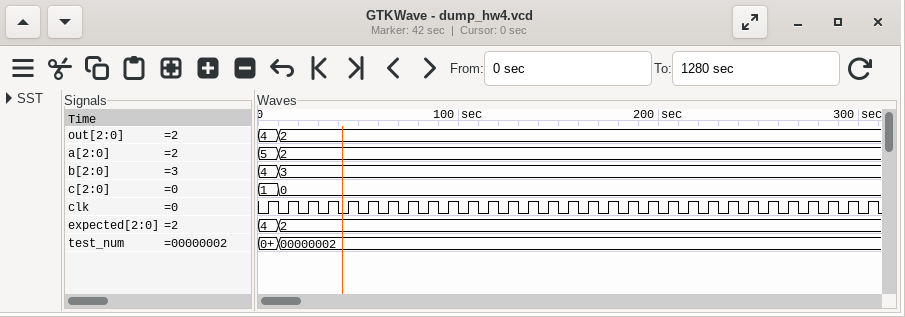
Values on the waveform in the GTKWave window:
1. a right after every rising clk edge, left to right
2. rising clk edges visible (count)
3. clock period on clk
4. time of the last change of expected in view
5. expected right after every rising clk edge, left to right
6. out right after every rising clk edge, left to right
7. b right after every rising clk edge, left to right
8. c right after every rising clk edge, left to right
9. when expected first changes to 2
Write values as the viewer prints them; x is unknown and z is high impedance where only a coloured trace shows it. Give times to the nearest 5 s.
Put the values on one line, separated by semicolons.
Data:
5, 2, 2, 2, 2, 2, 2, 2, 2, 2, 2, 2, 2, 2, 2, 2, 2, 2, 2, 2, 2, 2, 2, 2, 2, 2, 2, 2, 2, 2, 2; 31; 10 s; 10 s; 4, 2, 2, 2, 2, 2, 2, 2, 2, 2, 2, 2, 2, 2, 2, 2, 2, 2, 2, 2, 2, 2, 2, 2, 2, 2, 2, 2, 2, 2, 2; 4, 2, 2, 2, 2, 2, 2, 2, 2, 2, 2, 2, 2, 2, 2, 2, 2, 2, 2, 2, 2, 2, 2, 2, 2, 2, 2, 2, 2, 2, 2; 4, 3, 3, 3, 3, 3, 3, 3, 3, 3, 3, 3, 3, 3, 3, 3, 3, 3, 3, 3, 3, 3, 3, 3, 3, 3, 3, 3, 3, 3, 3; 1, 0, 0, 0, 0, 0, 0, 0, 0, 0, 0, 0, 0, 0, 0, 0, 0, 0, 0, 0, 0, 0, 0, 0, 0, 0, 0, 0, 0, 0, 0; 10 s
